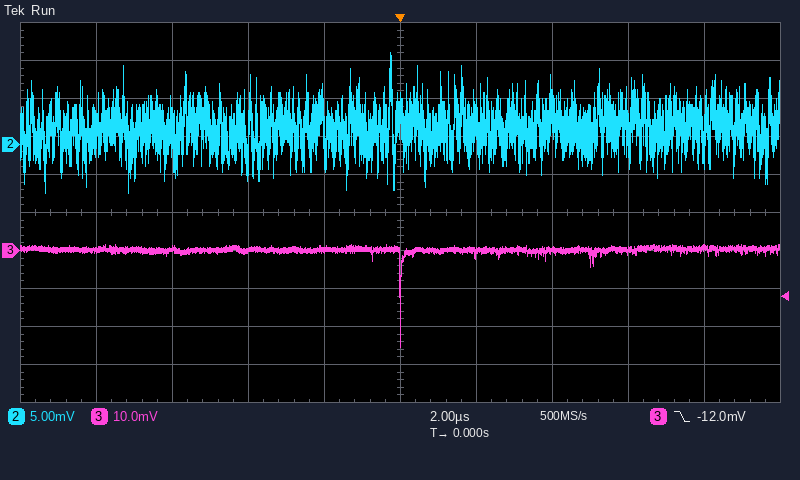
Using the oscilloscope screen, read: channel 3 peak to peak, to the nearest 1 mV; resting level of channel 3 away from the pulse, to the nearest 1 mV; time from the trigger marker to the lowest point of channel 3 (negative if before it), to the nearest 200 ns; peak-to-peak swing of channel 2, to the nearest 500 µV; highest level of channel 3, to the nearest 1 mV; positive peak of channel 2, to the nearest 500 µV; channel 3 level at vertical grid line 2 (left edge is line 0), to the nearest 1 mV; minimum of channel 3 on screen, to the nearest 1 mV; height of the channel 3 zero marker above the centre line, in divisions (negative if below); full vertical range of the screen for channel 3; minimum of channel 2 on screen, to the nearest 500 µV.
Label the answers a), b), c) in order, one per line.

a) 27 mV
b) 0 mV
c) 0.0 µs
d) 18.5 mV
e) 2 mV
f) 12.0 mV
g) 0 mV
h) -25 mV
i) -1.0 div
j) 100 mV
k) -6.5 mV
